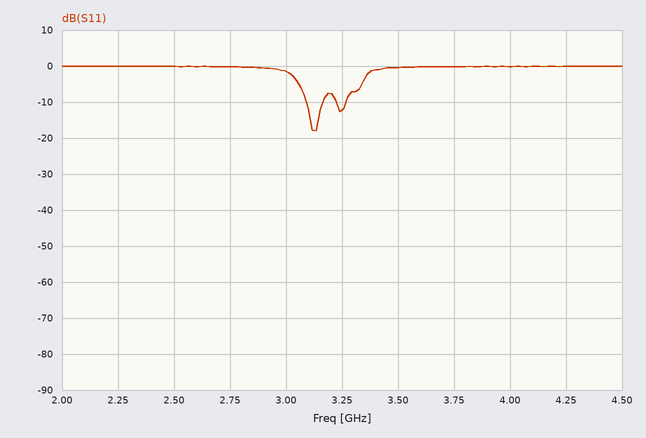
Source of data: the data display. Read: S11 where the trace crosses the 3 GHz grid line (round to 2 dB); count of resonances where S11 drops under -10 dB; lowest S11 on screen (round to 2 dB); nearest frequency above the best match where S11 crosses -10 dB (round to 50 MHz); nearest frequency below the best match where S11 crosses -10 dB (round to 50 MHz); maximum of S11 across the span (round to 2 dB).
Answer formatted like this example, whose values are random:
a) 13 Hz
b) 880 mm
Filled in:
a) -2 dB
b) 2
c) -18 dB
d) 3.15 GHz
e) 3.10 GHz
f) 0 dB
